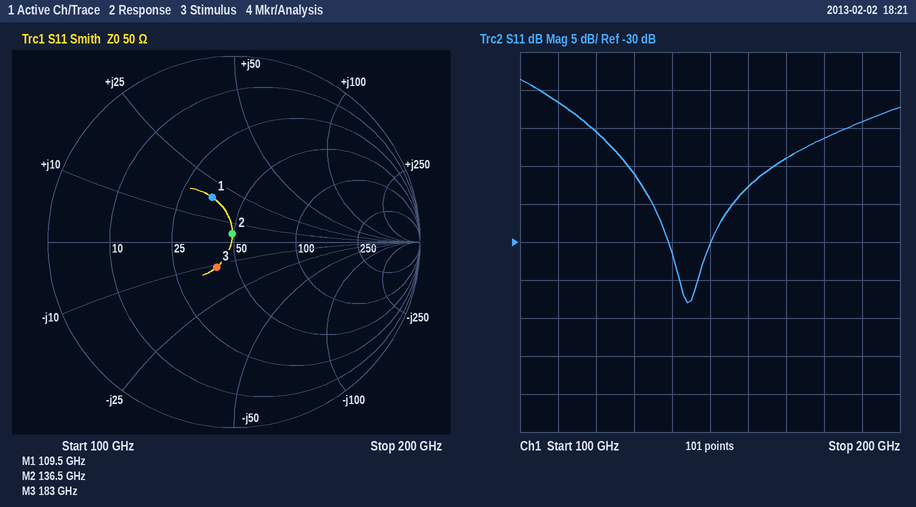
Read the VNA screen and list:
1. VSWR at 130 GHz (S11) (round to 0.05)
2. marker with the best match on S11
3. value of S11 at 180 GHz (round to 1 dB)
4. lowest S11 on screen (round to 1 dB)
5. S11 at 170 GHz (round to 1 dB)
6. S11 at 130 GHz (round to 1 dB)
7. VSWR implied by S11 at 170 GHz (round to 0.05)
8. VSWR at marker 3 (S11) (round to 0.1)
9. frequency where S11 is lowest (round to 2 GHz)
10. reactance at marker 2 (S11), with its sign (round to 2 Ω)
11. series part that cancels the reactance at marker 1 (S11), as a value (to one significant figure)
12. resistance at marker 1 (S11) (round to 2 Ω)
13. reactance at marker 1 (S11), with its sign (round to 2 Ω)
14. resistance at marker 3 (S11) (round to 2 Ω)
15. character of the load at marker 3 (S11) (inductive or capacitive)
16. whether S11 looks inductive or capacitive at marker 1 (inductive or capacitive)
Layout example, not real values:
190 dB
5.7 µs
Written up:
1.20
marker 2
-16 dB
-38 dB
-19 dB
-21 dB
1.25
1.4
144 GHz
+4 Ω
80 fF
36 Ω
+18 Ω
40 Ω
capacitive
inductive
